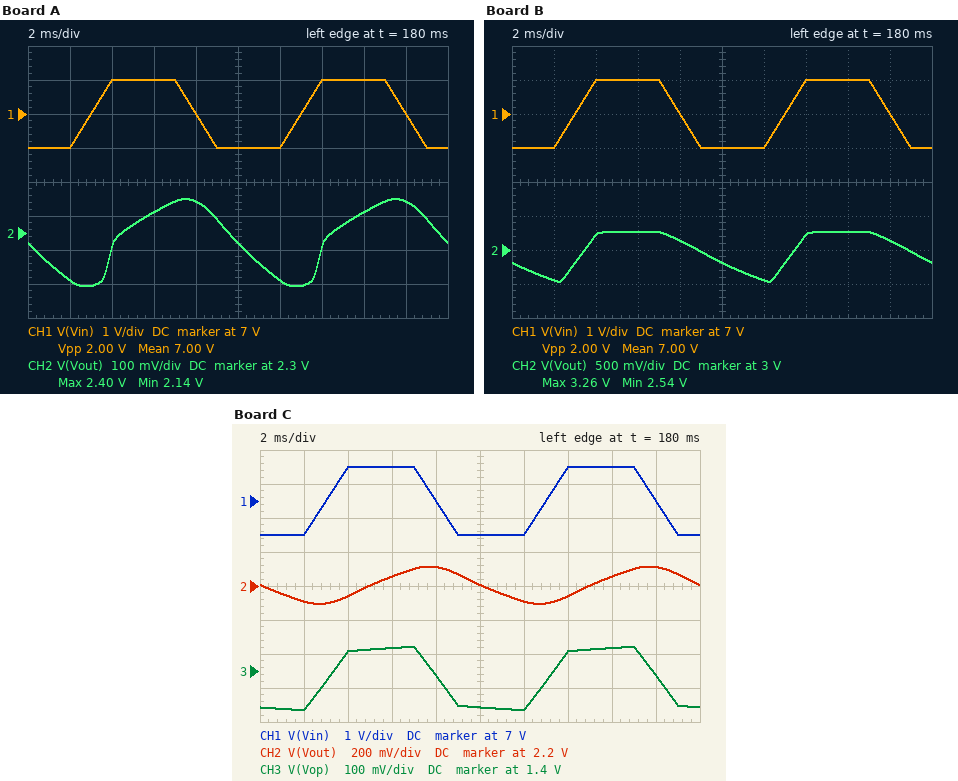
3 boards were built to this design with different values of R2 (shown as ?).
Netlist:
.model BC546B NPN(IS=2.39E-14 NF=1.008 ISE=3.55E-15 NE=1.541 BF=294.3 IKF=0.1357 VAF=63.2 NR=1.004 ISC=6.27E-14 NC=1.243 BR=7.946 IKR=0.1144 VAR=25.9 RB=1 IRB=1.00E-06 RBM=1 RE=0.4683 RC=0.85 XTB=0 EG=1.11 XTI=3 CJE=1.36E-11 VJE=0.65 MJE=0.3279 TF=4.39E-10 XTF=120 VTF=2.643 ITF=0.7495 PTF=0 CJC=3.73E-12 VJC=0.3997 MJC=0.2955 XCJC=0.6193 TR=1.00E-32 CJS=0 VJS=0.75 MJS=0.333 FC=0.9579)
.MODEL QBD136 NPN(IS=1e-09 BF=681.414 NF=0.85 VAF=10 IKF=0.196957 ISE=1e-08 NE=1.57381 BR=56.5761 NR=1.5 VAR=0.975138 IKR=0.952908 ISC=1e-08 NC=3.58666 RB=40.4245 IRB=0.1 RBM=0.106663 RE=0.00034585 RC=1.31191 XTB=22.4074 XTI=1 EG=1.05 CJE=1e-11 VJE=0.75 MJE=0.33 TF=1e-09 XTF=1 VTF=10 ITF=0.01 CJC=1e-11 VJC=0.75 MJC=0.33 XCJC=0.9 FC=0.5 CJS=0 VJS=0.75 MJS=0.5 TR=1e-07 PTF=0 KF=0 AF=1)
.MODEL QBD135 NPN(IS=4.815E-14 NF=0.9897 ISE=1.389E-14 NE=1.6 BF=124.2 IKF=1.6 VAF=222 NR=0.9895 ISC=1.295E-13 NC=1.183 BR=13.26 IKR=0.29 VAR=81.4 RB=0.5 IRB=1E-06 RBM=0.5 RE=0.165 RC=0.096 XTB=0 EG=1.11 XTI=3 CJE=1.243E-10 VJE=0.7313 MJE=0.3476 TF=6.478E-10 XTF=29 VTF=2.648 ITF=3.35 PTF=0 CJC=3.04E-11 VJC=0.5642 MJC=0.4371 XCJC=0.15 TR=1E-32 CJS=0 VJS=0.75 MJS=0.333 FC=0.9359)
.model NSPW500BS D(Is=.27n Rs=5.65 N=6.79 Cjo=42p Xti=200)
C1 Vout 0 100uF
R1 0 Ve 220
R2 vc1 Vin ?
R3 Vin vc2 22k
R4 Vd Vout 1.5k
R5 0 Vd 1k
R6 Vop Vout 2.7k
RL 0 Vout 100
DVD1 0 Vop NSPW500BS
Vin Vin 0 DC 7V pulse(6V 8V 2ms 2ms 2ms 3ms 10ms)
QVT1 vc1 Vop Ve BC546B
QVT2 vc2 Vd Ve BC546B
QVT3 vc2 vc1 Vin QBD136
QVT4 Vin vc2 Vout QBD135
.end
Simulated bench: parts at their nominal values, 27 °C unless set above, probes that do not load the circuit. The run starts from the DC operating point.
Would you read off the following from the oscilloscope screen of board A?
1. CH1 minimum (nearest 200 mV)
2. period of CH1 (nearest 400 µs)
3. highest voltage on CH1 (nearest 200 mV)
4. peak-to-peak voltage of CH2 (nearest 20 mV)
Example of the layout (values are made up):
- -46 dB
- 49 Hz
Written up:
- 6.0 V
- 10.0 ms
- 8.0 V
- 260 mV
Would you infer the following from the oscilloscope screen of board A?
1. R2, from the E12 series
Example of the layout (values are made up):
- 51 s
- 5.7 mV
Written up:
- 680 Ω
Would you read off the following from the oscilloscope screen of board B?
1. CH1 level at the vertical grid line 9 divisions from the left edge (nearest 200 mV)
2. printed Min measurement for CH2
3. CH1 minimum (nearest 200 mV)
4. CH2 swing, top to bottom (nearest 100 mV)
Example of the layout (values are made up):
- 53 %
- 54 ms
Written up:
- 7.0 V
- 2.54 V
- 6.0 V
- 700 mV
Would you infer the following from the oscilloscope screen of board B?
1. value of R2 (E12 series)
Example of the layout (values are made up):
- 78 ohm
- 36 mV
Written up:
- 330 Ω
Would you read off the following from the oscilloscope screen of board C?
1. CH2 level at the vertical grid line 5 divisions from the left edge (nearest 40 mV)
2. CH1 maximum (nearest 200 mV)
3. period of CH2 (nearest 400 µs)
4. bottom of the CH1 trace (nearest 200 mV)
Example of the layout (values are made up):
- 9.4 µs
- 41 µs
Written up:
- 2.20 V
- 8.0 V
- 10.0 ms
- 6.0 V
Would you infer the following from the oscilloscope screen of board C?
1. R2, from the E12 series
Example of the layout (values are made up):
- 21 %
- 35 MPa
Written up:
- 2.2 kΩ
